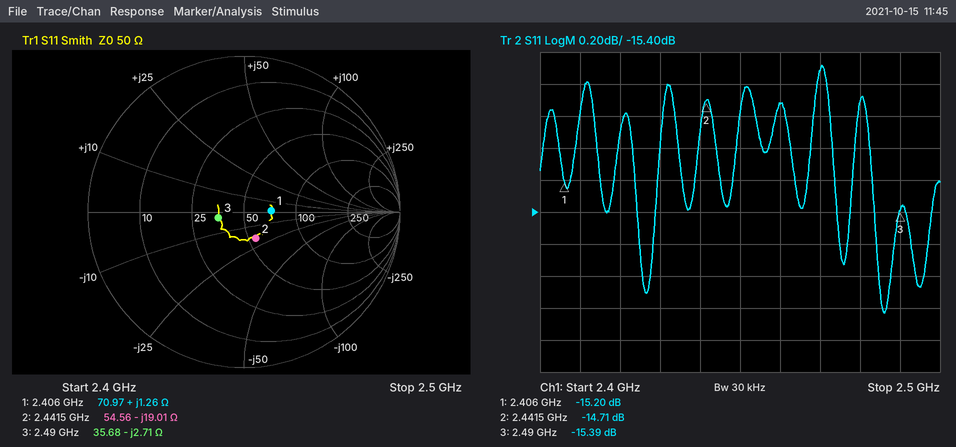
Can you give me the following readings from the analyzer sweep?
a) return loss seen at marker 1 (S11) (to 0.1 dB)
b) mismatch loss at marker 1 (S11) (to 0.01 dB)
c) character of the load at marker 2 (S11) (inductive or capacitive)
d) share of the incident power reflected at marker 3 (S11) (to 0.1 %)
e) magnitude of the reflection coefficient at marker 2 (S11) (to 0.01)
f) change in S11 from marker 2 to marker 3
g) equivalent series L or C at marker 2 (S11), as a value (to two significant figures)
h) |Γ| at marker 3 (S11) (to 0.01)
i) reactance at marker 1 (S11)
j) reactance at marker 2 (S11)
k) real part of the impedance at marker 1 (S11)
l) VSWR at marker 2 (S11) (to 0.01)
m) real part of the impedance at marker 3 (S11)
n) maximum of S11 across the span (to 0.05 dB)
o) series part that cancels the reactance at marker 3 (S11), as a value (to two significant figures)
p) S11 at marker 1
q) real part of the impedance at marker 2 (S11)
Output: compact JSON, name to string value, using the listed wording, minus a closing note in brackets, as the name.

{"return loss seen at marker 1 (S11)": "15.2 dB", "mismatch loss at marker 1 (S11)": "0.13 dB", "character of the load at marker 2 (S11)": "capacitive", "share of the incident power reflected at marker 3 (S11)": "2.9 %", "magnitude of the reflection coefficient at marker 2 (S11)": "0.18", "change in S11 from marker 2 to marker 3": "-0.68 dB", "equivalent series L or C at marker 2 (S11), as a value": "3.4 pF", "|Γ| at marker 3 (S11)": "0.17", "reactance at marker 1": "+1.26 Ω", "reactance at marker 2": "-19.01 Ω", "real part of the impedance at marker 1": "70.97 Ω", "VSWR at marker 2 (S11)": "1.45", "real part of the impedance at marker 3": "35.68 Ω", "maximum of S11 across the span": "-14.50 dB", "series part that cancels the reactance at marker 3 (S11), as a value": "170 pH", "S11 at marker 1": "-15.20 dB", "real part of the impedance at marker 2": "54.56 Ω"}
